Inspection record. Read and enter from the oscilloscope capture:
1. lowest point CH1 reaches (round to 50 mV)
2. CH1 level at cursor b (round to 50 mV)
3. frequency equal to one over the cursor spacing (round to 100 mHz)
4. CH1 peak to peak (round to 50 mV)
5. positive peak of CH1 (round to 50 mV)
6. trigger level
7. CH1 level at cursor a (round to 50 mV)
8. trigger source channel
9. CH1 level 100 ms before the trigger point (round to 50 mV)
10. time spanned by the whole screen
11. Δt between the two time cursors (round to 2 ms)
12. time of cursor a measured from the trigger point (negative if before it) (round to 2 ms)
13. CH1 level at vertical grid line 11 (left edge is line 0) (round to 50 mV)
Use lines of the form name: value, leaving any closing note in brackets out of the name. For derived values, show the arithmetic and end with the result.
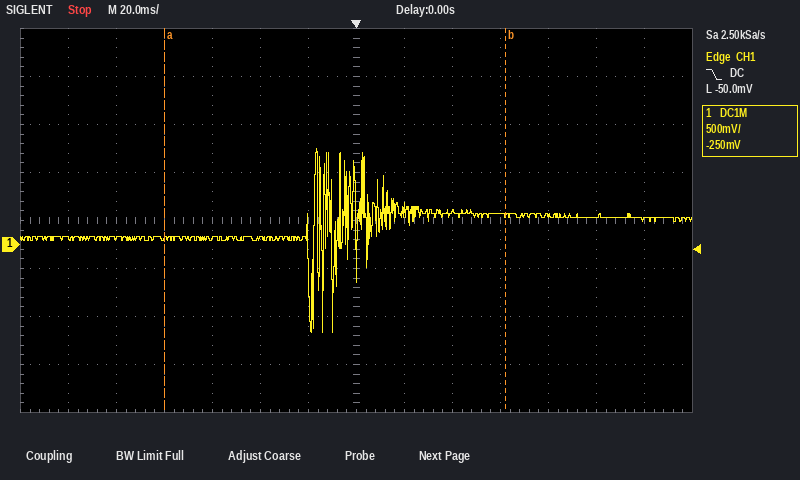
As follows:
lowest point CH1 reaches: -900 mV
CH1 level at cursor b: 300 mV
frequency equal to one over the cursor spacing: 1 / 142 ms ≈ 7.0 Hz
CH1 peak to peak: 1.00 V − (-900 mV) = 1.90 V
positive peak of CH1: 1.00 V
trigger level: -50.0 mV
CH1 level at cursor a: 50 mV
trigger source channel: CH1
CH1 level 100 ms before the trigger point: 50 mV
time spanned by the whole screen: 280 ms
Δt between the two time cursors: 142 ms
time of cursor a measured from the trigger point (negative if before it): -80 ms
CH1 level at vertical grid line 11 (left edge is line 0): 300 mV
